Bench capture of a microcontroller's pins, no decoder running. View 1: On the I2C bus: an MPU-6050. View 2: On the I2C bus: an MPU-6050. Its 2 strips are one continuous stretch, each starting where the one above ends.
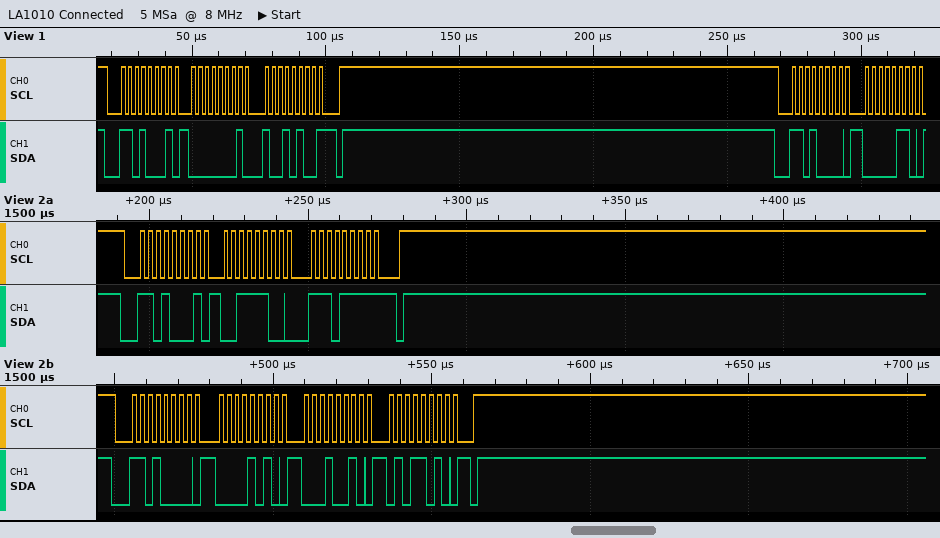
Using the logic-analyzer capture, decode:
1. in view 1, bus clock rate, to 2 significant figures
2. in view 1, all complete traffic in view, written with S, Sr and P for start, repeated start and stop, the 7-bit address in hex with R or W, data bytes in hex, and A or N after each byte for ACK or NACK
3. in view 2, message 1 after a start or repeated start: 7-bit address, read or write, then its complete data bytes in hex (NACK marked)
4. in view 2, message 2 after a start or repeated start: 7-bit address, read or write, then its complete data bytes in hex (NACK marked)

400 kHz
S 68R A 01 A 94 N P S 68W A 06 A
0x68 read: 3C EF NACK
0x68 write: 0A 12 5A
